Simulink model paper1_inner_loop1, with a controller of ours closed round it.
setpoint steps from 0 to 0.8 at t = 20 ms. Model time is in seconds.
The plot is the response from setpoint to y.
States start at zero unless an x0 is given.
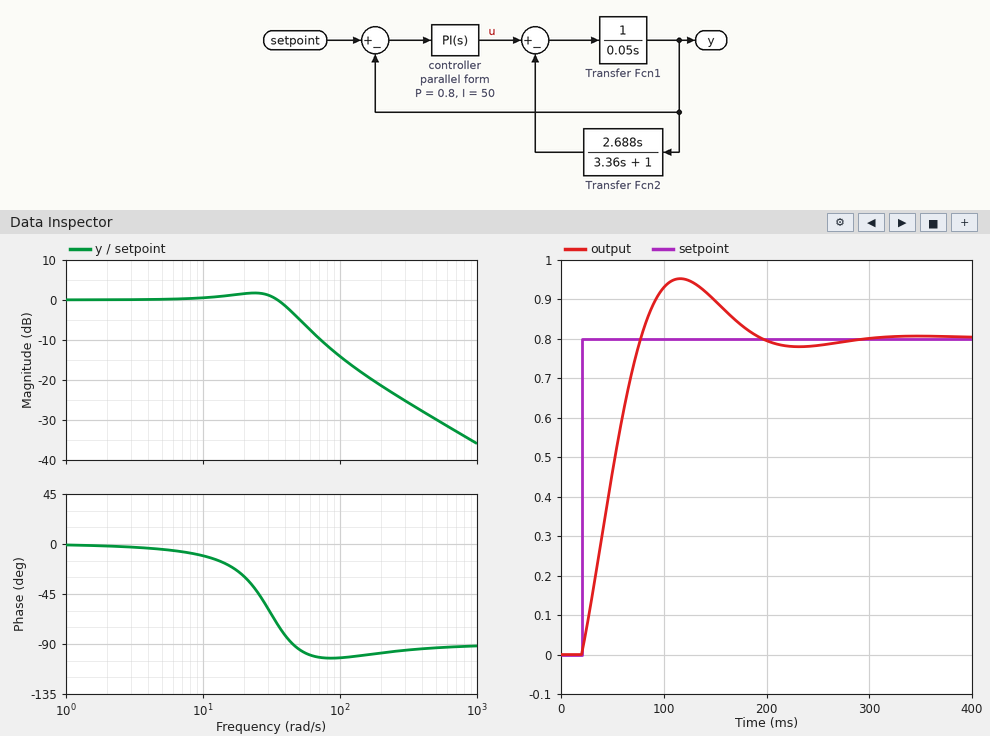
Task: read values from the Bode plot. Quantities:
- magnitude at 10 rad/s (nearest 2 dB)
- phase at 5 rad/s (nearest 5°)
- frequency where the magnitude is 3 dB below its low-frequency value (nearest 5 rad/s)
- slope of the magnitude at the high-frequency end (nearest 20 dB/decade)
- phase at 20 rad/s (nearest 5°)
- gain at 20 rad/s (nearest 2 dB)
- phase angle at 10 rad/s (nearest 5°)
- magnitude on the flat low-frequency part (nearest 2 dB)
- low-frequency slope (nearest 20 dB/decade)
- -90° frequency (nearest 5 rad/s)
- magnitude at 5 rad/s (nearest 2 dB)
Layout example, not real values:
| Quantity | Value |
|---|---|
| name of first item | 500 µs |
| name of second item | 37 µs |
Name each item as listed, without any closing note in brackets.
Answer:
| Quantity | Value |
|---|---|
| magnitude at 10 rad/s | 0 dB |
| phase at 5 rad/s | -5° |
| frequency where the magnitude is 3 dB below its low-frequency value | 45 rad/s |
| slope of the magnitude at the high-frequency end | -20 dB/decade |
| phase at 20 rad/s | -30° |
| gain at 20 rad/s | 2 dB |
| phase angle at 10 rad/s | -10° |
| magnitude on the flat low-frequency part | 0 dB |
| low-frequency slope | 0 dB/decade |
| -90° frequency | 45 rad/s |
| magnitude at 5 rad/s | 0 dB |
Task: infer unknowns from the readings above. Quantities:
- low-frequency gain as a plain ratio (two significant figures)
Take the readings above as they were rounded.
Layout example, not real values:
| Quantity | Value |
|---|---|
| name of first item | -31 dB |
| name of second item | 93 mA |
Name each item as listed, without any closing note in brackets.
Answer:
| Quantity | Value |
|---|---|
| low-frequency gain as a plain ratio | 1.0 |
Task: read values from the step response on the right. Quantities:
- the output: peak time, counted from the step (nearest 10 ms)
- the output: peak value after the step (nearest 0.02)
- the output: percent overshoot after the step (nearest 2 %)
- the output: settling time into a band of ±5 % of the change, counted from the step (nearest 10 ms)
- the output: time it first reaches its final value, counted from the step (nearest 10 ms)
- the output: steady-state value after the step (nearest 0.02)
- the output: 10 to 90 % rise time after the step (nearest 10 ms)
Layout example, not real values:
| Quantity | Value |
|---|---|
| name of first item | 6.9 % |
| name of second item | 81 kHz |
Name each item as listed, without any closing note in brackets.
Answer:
| Quantity | Value |
|---|---|
| the output: peak time, counted from the step | 100 ms |
| the output: peak value after the step | 0.96 |
| the output: percent overshoot after the step | 18 % |
| the output: settling time into a band of ±5 % of the change, counted from the step | 150 ms |
| the output: time it first reaches its final value, counted from the step | 60 ms |
| the output: steady-state value after the step | 0.80 |
| the output: 10 to 90 % rise time after the step | 40 ms |
